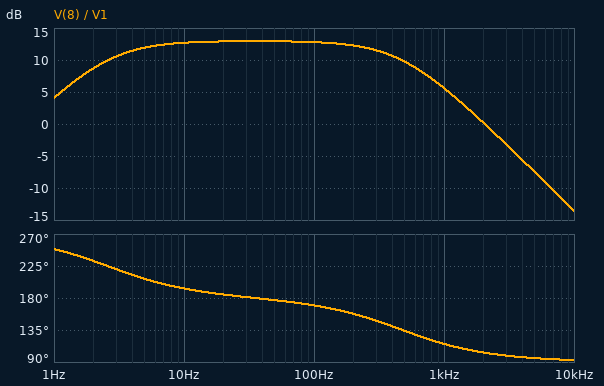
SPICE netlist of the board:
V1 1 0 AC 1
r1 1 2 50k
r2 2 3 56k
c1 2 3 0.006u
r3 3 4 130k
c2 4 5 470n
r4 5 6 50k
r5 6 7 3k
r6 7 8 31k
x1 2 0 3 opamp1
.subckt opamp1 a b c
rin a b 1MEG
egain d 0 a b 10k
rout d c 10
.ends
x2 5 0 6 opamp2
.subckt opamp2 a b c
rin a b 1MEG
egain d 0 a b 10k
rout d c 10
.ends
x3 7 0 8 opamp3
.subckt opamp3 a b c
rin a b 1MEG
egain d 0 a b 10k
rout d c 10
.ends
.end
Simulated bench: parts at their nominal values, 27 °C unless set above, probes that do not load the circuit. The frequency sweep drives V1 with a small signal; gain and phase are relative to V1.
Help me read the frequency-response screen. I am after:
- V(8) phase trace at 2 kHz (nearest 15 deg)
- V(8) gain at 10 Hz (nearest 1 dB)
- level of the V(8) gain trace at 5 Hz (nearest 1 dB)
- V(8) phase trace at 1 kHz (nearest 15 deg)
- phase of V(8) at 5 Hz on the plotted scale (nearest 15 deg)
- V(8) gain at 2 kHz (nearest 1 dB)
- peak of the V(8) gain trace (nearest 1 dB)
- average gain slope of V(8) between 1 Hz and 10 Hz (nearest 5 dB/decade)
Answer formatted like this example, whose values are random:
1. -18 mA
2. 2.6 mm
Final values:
1. 105 deg
2. 13 dB
3. 12 dB
4. 120 deg
5. 210 deg
6. 0 dB
7. 13 dB
8. 10 dB/decade
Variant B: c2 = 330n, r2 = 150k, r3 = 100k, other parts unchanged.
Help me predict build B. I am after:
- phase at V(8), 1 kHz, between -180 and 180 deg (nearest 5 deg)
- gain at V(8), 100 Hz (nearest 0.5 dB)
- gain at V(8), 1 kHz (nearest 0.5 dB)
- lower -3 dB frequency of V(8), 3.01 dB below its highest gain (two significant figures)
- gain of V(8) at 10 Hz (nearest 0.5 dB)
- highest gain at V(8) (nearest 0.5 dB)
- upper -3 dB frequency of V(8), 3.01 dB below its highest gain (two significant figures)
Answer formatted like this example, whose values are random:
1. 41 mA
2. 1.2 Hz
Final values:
1. 100 deg
2. 22.5 dB
3. 8.5 dB
4. 4.6 Hz
5. 23.0 dB
6. 23.5 dB
7. 190 Hz
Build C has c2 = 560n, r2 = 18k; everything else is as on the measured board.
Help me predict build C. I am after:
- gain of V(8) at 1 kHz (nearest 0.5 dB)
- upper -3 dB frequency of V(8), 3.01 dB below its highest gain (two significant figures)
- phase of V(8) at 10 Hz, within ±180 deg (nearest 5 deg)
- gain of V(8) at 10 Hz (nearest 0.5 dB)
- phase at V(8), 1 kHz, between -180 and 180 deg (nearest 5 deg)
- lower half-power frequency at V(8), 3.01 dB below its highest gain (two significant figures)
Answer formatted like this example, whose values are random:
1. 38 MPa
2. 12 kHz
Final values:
1. 1.5 dB
2. 1.5 kHz
3. -170 deg
4. 3.0 dB
5. 145 deg
6. 2.2 Hz
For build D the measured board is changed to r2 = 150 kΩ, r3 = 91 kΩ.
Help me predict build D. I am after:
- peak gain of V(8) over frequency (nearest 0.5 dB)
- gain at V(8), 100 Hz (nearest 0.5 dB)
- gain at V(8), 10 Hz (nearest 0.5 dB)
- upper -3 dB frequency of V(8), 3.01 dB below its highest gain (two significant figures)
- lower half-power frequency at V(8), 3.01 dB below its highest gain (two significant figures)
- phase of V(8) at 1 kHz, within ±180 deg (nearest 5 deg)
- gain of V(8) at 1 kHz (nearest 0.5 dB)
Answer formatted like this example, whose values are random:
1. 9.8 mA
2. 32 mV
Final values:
1. 24.5 dB
2. 23.5 dB
3. 24.0 dB
4. 180 Hz
5. 3.6 Hz
6. 100 deg
7. 9.5 dB
